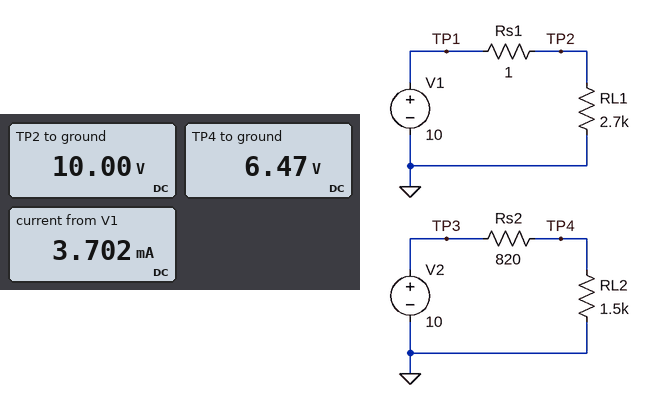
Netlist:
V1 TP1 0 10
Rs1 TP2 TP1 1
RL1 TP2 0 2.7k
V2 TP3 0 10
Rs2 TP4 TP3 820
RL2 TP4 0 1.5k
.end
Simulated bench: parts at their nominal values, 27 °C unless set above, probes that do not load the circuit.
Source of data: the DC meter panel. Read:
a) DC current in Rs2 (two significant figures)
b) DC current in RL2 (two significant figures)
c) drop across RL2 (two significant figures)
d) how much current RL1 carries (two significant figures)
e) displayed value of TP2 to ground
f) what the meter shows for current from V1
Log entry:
4.3 mA
4.3 mA
6.5 V
3.7 mA
10.00 V
3.702 mA
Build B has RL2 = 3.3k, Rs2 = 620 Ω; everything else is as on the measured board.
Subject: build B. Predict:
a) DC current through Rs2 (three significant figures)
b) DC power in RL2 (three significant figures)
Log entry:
2.55 mA
21.5 mW
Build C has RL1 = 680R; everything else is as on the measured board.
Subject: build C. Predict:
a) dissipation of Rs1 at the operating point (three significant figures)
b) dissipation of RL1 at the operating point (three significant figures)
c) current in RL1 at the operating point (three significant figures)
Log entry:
216 µW
147 mW
14.7 mA
